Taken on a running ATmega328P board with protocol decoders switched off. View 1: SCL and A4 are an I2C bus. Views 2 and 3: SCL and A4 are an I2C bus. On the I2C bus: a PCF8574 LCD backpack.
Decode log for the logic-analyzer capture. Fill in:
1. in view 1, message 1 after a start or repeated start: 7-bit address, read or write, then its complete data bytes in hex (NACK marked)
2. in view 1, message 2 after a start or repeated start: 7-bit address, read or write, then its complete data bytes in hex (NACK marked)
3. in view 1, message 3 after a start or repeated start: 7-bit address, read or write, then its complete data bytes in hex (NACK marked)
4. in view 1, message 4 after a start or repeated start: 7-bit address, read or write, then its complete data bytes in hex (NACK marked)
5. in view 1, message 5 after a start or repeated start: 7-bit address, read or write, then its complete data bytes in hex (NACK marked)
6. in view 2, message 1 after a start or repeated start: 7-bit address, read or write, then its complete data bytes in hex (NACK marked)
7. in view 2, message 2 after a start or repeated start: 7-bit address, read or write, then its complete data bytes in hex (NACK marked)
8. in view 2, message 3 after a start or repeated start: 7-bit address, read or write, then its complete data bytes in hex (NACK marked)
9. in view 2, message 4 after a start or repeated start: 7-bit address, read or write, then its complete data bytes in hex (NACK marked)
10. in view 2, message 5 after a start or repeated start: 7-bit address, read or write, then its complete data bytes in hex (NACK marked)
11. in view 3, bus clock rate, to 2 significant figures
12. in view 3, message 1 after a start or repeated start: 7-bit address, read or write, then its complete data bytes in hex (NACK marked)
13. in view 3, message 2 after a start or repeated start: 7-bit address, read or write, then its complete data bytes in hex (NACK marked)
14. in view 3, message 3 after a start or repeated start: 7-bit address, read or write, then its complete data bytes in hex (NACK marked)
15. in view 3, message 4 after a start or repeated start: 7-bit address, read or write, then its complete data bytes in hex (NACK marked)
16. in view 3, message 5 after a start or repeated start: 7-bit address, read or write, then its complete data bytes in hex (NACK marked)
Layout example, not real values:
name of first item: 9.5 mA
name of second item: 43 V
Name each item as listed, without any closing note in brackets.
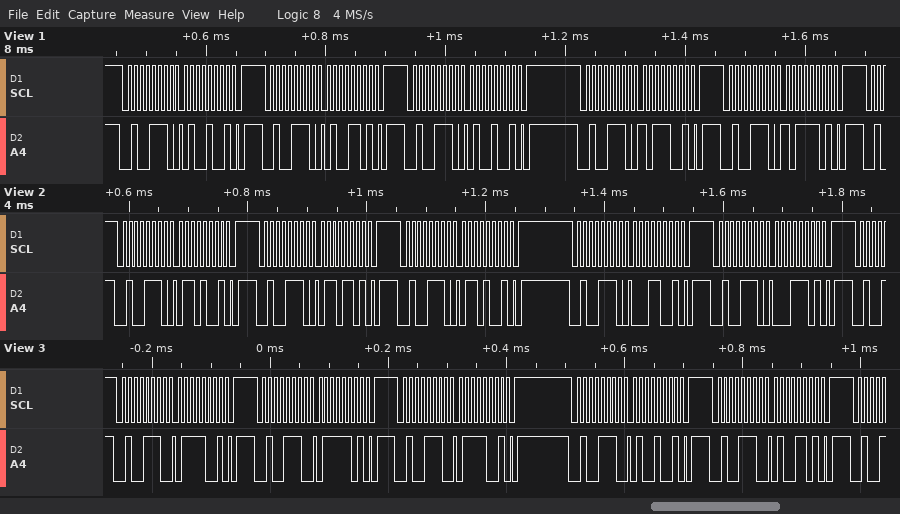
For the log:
in view 1, message 1 after a start or repeated start: 7-bit address, read or write, then its complete data bytes in hex: 0x27 write: 49
in view 1, message 2 after a start or repeated start: 7-bit address, read or write, then its complete data bytes in hex: 0x27 write: 4D
in view 1, message 3 after a start or repeated start: 7-bit address, read or write, then its complete data bytes in hex: 0x27 write: 49
in view 1, message 4 after a start or repeated start: 7-bit address, read or write, then its complete data bytes in hex: 0x27 write: B9
in view 1, message 5 after a start or repeated start: 7-bit address, read or write, then its complete data bytes in hex: 0x27 write: BD
in view 2, message 1 after a start or repeated start: 7-bit address, read or write, then its complete data bytes in hex: 0x27 write: 69
in view 2, message 2 after a start or repeated start: 7-bit address, read or write, then its complete data bytes in hex: 0x27 write: 6D
in view 2, message 3 after a start or repeated start: 7-bit address, read or write, then its complete data bytes in hex: 0x27 write: 69
in view 2, message 4 after a start or repeated start: 7-bit address, read or write, then its complete data bytes in hex: 0x27 write: 19
in view 2, message 5 after a start or repeated start: 7-bit address, read or write, then its complete data bytes in hex: 0x27 write: 1D
in view 3, bus clock rate, to 2 significant figures: 100 kHz
in view 3, message 1 after a start or repeated start: 7-bit address, read or write, then its complete data bytes in hex: 0x27 write: 79
in view 3, message 2 after a start or repeated start: 7-bit address, read or write, then its complete data bytes in hex: 0x27 write: 7D
in view 3, message 3 after a start or repeated start: 7-bit address, read or write, then its complete data bytes in hex: 0x27 write: 79
in view 3, message 4 after a start or repeated start: 7-bit address, read or write, then its complete data bytes in hex: 0x27 write: 49
in view 3, message 5 after a start or repeated start: 7-bit address, read or write, then its complete data bytes in hex: 0x27 write: 4D
